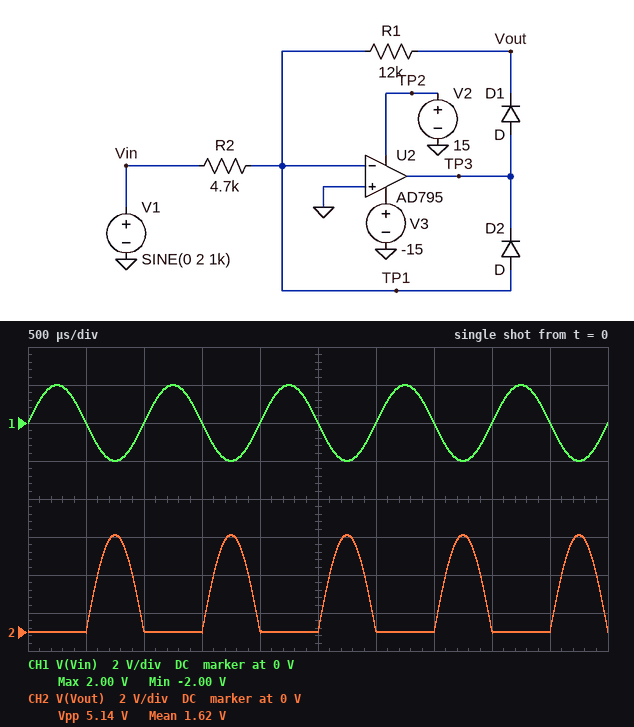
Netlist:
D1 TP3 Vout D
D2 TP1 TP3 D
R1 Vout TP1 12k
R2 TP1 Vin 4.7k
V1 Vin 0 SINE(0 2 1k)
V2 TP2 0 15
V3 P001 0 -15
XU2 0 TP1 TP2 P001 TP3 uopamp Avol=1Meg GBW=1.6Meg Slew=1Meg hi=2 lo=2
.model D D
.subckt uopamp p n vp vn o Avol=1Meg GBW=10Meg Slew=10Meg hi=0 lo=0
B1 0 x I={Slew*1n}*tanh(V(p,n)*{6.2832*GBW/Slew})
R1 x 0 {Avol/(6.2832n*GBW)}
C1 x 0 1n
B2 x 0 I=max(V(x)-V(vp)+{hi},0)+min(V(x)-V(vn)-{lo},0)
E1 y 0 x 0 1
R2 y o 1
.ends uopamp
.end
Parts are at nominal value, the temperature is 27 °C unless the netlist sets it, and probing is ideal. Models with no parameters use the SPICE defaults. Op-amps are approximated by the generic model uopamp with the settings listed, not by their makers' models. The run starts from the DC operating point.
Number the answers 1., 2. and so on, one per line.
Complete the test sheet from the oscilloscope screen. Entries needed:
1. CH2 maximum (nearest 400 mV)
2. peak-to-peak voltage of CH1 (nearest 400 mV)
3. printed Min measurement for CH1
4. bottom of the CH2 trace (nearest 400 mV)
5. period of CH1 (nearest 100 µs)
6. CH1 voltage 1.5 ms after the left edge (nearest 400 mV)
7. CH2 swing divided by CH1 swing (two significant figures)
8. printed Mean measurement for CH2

1. 5.2 V
2. 4.0 V
3. -2.00 V
4. 0 V
5. 1.0 ms
6. 0 V
7. 1.3
8. 1.62 V
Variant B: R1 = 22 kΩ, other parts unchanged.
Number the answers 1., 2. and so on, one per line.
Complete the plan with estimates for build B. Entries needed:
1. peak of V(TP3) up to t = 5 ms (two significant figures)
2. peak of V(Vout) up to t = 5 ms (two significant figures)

1. 10 V
2. 9.4 V
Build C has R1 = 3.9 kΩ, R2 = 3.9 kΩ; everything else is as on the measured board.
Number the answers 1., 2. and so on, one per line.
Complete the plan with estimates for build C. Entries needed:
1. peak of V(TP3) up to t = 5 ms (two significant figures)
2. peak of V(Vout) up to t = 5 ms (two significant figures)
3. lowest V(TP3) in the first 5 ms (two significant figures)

1. 2.6 V
2. 2.0 V
3. -640 mV
